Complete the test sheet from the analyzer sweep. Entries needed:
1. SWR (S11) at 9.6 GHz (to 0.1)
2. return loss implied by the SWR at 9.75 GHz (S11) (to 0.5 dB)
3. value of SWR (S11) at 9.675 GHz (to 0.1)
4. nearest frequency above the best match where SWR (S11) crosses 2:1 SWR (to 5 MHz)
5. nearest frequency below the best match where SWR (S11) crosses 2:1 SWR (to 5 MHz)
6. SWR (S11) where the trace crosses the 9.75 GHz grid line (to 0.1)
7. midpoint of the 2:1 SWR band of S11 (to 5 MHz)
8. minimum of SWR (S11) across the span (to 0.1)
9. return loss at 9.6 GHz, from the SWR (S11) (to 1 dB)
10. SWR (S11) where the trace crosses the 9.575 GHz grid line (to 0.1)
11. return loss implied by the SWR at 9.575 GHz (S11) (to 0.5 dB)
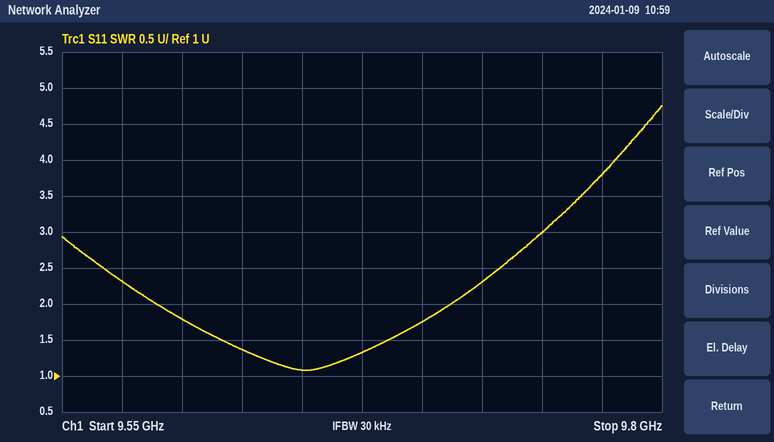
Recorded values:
1.8
6.0 dB
1.3
9.710 GHz
9.590 GHz
3.0
9.650 GHz
1.1
11 dB
2.3
8.0 dB
